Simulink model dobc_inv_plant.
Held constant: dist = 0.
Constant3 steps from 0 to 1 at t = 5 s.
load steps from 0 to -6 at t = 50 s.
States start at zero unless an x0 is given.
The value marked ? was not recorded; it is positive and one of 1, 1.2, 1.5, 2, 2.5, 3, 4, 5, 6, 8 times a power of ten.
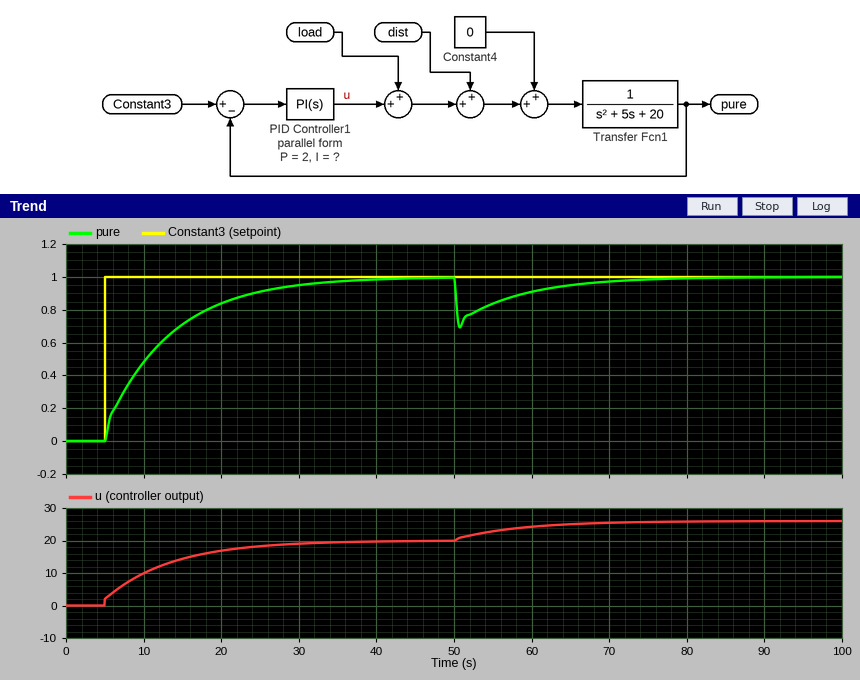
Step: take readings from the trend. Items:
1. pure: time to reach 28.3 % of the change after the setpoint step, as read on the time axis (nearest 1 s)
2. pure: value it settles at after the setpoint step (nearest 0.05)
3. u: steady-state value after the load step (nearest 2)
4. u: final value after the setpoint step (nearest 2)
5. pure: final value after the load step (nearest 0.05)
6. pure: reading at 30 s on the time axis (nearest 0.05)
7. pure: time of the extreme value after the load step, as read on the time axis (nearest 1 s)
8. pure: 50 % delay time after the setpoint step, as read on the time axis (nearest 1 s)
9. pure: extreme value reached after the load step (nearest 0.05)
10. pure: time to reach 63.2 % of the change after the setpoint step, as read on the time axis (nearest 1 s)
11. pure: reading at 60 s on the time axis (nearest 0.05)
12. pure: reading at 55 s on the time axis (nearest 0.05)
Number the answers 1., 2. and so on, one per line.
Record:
1. 7 s
2. 1.00
3. 26
4. 20
5. 1.00
6. 0.95
7. 51 s
8. 10 s
9. 0.70
10. 13 s
11. 0.90
12. 0.85
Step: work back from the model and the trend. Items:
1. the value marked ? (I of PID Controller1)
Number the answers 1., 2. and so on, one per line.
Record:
1. 2.5
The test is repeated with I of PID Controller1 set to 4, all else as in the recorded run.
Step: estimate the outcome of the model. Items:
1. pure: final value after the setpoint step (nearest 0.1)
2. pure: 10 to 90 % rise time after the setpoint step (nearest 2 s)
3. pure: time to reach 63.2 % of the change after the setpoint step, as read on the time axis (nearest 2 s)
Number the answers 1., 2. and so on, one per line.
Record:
1. 1.0
2. 12 s
3. 10 s
